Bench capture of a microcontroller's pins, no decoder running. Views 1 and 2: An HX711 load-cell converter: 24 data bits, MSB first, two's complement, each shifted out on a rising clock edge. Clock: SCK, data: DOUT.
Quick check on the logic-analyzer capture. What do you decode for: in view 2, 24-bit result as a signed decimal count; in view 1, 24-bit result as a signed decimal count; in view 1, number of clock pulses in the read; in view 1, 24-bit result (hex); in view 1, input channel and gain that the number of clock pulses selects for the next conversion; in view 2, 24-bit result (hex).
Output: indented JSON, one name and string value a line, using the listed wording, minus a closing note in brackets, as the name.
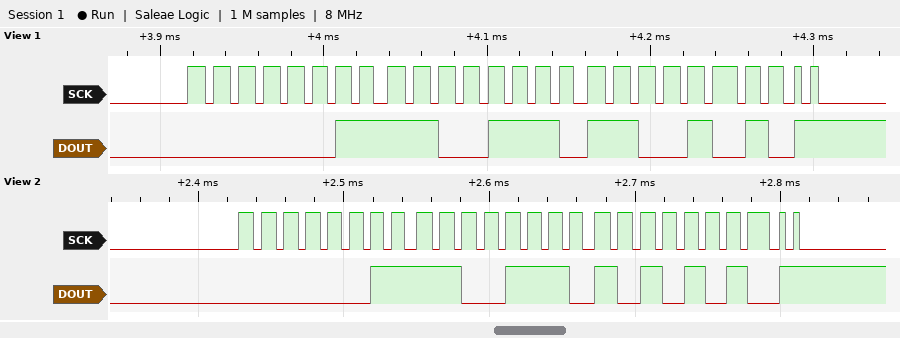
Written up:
{
  "in view 2, 24-bit result as a signed decimal count": "249514",
  "in view 1, 24-bit result as a signed decimal count": "249546",
  "in view 1, number of clock pulses in the read": "26",
  "in view 1, 24-bit result": "0x03CECA",
  "in view 1, input channel and gain that the number of clock pulses selects for the next conversion": "channel B, gain 32",
  "in view 2, 24-bit result": "0x03CEAA"
}
